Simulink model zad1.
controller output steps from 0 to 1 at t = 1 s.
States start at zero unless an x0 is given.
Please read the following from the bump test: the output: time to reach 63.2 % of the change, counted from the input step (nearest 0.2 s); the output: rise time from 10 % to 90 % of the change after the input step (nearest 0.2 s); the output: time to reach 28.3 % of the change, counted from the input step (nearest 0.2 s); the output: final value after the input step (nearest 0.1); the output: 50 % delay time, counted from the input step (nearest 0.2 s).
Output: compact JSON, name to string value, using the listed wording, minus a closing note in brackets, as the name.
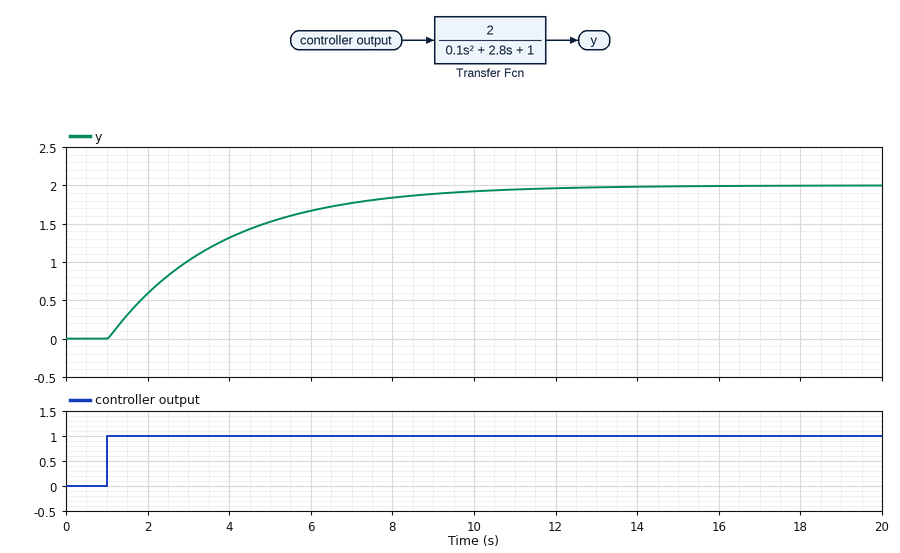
{"the output: time to reach 63.2 % of the change, counted from the input step": "2.8 s", "the output: rise time from 10 % to 90 % of the change after the input step": "6.0 s", "the output: time to reach 28.3 % of the change, counted from the input step": "1.0 s", "the output: final value after the input step": "2.0", "the output: 50 % delay time, counted from the input step": "2.0 s"}
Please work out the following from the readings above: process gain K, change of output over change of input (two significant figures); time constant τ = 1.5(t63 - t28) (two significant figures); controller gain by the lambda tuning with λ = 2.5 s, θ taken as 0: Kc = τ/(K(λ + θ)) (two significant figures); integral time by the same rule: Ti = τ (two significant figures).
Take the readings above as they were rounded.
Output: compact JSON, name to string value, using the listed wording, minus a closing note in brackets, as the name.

{"process gain K, change of output over change of input": "2.0", "time constant τ = 1.5(t63 - t28)": "2.7 s", "controller gain by the lambda tuning with λ = 2.5 s, θ taken as 0: Kc = τ/(K(λ + θ))": "0.54", "integral time by the same rule: Ti = τ": "2.7 s"}
